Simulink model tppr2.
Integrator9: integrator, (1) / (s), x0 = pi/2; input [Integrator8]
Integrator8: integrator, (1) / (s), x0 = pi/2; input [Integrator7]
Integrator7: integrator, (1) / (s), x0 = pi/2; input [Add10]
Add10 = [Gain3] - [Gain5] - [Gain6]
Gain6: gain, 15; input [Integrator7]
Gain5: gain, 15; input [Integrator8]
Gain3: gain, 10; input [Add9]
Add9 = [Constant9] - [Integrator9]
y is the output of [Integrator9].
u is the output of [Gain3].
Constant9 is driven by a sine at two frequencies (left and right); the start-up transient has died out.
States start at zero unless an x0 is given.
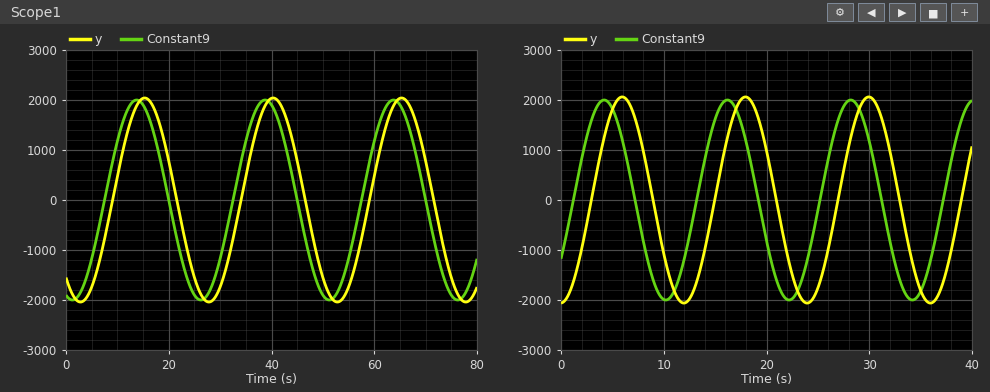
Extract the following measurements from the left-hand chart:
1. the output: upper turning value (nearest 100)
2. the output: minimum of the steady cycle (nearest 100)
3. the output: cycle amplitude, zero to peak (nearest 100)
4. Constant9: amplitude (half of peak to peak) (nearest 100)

2000
-2000
2000
2000
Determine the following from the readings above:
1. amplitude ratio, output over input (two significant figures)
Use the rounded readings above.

1.0
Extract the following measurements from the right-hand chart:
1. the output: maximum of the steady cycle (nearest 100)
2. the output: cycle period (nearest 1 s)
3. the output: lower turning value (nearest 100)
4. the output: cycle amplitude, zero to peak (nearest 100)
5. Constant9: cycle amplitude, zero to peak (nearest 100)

2100
12 s
-2100
2100
2000
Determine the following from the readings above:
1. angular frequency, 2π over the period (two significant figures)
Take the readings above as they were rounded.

0.52 rad/s
